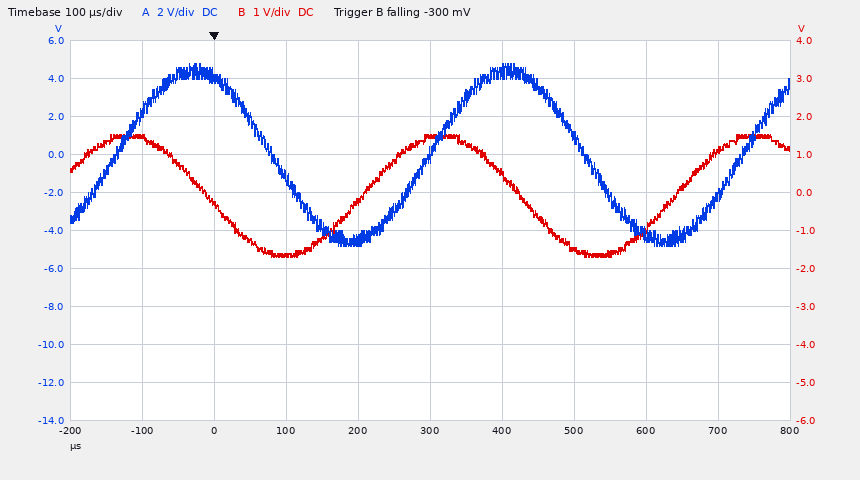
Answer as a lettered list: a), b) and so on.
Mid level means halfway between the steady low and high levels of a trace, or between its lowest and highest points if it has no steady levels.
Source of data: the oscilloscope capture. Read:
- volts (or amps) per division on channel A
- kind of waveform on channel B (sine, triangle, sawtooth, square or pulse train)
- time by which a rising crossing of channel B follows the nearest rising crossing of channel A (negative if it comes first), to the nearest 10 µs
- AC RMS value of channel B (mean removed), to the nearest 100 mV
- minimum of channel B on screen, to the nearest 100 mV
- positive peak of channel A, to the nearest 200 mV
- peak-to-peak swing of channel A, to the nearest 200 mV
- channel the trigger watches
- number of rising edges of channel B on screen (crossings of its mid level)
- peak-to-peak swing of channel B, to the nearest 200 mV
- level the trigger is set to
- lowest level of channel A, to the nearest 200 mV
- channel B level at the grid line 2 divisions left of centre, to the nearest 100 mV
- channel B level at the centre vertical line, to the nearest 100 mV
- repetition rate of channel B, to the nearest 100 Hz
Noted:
a) 2 V
b) sine
c) -90 µs
d) 1.1 V
e) -1.7 V
f) 4.8 V
g) 9.6 V
h) channel B
i) 2
j) 3.2 V
k) -300 mV
l) -4.8 V
m) -1.6 V
n) 1.5 V
o) 2.3 kHz
